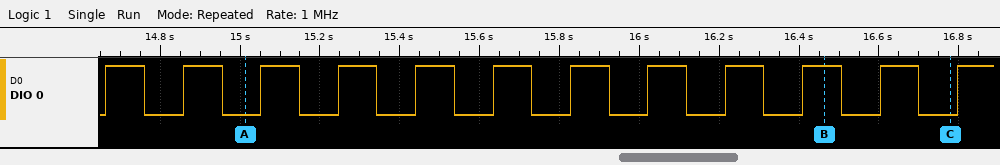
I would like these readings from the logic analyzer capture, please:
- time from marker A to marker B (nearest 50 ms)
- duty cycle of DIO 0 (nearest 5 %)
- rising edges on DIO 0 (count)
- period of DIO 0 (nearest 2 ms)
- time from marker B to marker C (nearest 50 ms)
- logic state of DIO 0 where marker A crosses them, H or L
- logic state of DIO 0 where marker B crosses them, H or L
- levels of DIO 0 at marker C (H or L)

1450 ms
50 %
12
194 ms
300 ms
DIO 0=L
DIO 0=H
DIO 0=L
